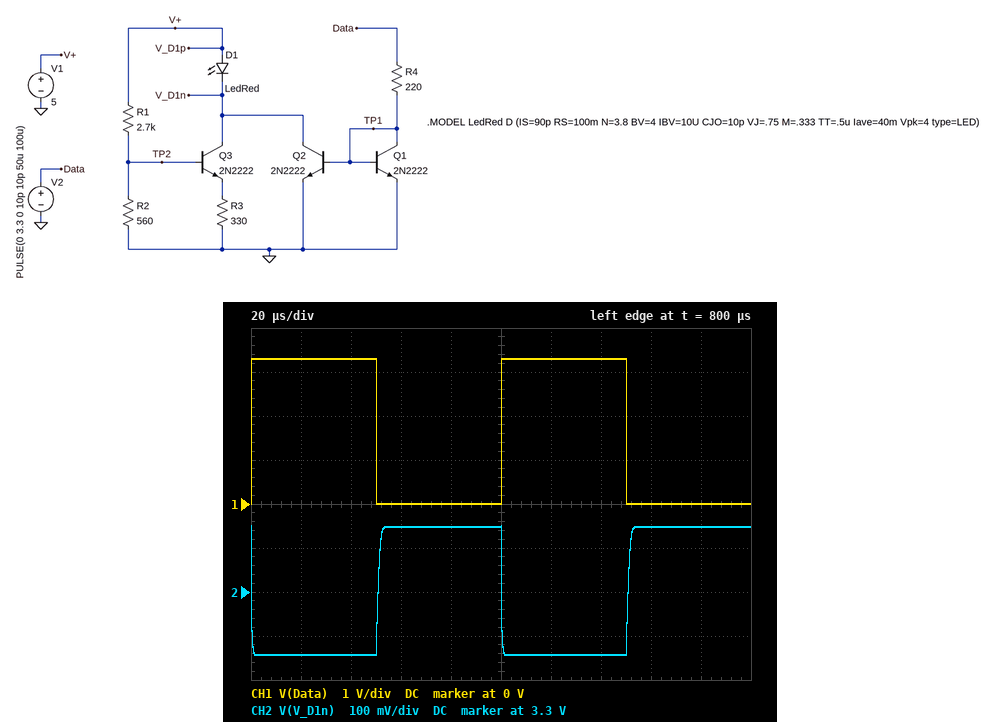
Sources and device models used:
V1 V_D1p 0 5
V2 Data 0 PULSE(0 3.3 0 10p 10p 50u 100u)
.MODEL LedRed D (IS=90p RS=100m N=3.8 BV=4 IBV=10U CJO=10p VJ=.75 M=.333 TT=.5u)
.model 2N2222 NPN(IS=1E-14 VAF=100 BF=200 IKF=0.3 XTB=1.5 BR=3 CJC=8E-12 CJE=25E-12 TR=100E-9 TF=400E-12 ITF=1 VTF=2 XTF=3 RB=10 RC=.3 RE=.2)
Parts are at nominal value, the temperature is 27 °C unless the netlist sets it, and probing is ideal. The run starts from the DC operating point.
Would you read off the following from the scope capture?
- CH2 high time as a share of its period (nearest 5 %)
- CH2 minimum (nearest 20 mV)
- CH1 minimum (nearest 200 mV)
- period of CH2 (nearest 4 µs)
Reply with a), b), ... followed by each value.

a) 50 %
b) 3.16 V
c) 0 V
d) 100 µs
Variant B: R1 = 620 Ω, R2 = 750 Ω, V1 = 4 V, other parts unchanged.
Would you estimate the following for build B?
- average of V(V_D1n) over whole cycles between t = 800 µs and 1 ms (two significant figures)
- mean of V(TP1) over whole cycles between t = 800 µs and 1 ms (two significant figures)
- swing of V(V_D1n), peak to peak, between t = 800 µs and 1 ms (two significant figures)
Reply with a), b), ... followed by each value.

a) 2.2 V
b) 360 mV
c) 130 mV
